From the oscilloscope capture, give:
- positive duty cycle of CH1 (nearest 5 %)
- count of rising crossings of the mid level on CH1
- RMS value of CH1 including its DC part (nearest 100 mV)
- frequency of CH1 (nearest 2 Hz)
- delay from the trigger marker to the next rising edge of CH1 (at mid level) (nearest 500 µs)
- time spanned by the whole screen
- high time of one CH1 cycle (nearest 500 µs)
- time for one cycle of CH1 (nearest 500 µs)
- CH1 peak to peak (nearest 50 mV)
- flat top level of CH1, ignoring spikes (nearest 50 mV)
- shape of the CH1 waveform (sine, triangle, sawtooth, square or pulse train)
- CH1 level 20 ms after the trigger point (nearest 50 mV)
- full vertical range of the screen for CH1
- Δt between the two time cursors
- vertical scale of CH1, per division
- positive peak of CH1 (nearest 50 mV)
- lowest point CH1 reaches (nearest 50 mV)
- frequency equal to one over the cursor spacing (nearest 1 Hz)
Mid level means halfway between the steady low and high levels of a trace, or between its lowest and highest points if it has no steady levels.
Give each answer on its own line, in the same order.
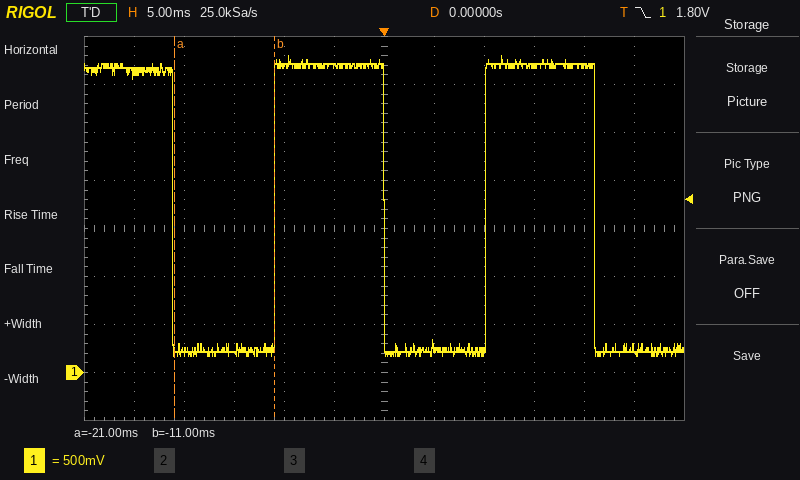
50 %
2
2.3 V
48 Hz
10.0 ms
60 ms
11.0 ms
21.0 ms
3.10 V
3.20 V
square
3.20 V
4 V
10.0 ms
500 mV
3.30 V
200 mV
100 Hz
